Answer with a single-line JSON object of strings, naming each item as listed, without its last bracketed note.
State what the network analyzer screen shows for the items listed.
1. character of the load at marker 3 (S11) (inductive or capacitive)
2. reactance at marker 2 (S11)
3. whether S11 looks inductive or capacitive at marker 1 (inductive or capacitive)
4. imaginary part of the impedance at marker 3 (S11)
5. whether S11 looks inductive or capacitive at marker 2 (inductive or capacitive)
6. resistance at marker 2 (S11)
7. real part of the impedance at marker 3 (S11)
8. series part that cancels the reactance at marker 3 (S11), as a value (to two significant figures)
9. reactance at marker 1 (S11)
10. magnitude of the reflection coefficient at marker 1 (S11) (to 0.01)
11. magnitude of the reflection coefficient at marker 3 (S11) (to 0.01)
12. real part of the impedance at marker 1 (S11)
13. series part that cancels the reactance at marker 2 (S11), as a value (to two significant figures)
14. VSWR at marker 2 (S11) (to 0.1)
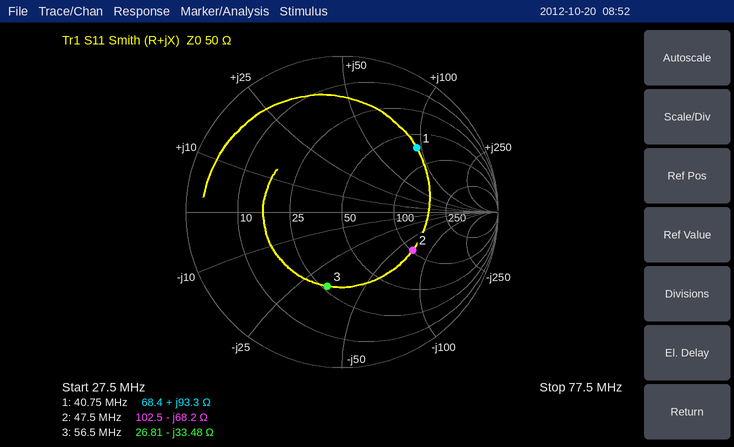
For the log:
{"character of the load at marker 3 (S11)": "capacitive", "reactance at marker 2": "-68.2 Ω", "whether S11 looks inductive or capacitive at marker 1": "inductive", "imaginary part of the impedance at marker 3": "-33.48 Ω", "whether S11 looks inductive or capacitive at marker 2": "capacitive", "resistance at marker 2": "102.5 Ω", "real part of the impedance at marker 3": "26.81 Ω", "series part that cancels the reactance at marker 3 (S11), as a value": "94 nH", "reactance at marker 1": "+93.3 Ω", "magnitude of the reflection coefficient at marker 1 (S11)": "0.63", "magnitude of the reflection coefficient at marker 3 (S11)": "0.49", "real part of the impedance at marker 1": "68.4 Ω", "series part that cancels the reactance at marker 2 (S11), as a value": "230 nH", "VSWR at marker 2 (S11)": "3.1"}
